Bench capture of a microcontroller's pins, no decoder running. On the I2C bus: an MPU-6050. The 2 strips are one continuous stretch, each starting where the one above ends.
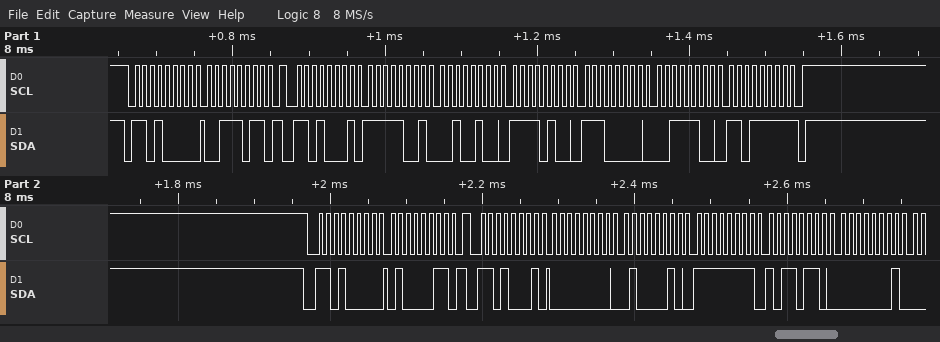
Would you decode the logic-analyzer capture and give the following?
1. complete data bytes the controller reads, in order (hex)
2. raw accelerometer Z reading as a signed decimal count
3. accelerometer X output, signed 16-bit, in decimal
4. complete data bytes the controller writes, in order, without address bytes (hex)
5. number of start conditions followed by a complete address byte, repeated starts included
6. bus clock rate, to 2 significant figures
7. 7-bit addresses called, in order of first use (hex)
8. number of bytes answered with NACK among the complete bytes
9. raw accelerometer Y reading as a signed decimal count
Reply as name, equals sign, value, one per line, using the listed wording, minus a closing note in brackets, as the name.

complete data bytes the controller reads, in order = F9 24 F4 E0 3C DF 00 42 FF B6 01
raw accelerometer Z reading as a signed decimal count = 15583
accelerometer X output, signed 16-bit, in decimal = -1756
complete data bytes the controller writes, in order, without address bytes = 3B 43
number of start conditions followed by a complete address byte, repeated starts included = 4
bus clock rate, to 2 significant figures = 100 kHz
7-bit addresses called, in order of first use = 0x68
number of bytes answered with NACK among the complete bytes = 1
raw accelerometer Y reading as a signed decimal count = -2848
